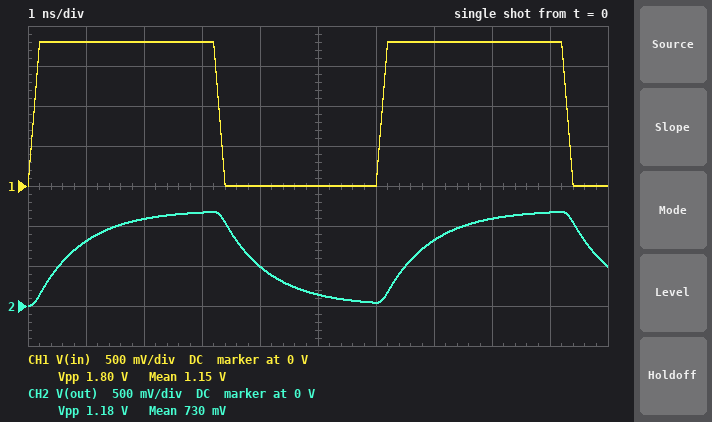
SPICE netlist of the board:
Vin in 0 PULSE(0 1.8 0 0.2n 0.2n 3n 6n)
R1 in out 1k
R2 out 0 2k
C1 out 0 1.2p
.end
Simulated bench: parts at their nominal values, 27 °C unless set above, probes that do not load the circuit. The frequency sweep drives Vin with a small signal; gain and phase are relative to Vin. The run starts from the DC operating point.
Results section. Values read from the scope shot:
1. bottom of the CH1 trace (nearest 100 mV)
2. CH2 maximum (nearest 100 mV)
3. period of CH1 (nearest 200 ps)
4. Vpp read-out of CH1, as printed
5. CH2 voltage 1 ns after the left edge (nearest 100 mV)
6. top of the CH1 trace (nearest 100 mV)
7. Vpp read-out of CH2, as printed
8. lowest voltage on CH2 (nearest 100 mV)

0 V
1.2 V
6.0 ns
1.80 V
800 mV
1.8 V
1.18 V
0 V
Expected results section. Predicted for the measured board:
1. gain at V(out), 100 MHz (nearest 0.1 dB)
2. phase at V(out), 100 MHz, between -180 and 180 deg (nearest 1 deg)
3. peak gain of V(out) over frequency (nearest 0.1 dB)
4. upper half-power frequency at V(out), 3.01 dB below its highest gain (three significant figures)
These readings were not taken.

-4.5 dB
-27 deg
-3.5 dB
199 MHz
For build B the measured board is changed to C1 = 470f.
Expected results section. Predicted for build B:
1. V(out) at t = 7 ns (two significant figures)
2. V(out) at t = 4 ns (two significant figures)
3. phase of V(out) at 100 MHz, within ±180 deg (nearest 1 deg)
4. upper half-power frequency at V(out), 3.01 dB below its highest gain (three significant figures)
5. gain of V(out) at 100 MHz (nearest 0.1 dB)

1.1 V
130 mV
-11 deg
508 MHz
-3.7 dB
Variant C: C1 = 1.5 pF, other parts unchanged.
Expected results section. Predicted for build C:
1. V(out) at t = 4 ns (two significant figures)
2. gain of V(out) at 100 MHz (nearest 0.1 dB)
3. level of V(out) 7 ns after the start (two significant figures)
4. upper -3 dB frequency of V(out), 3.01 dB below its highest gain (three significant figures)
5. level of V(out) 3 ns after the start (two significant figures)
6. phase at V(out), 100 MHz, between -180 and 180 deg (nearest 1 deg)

570 mV
-5.0 dB
740 mV
159 MHz
1.1 V
-32 deg
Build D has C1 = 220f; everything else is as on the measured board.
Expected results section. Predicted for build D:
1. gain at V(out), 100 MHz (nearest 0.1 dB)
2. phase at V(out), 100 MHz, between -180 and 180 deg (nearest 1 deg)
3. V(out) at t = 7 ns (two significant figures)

-3.6 dB
-5 deg
1.2 V
